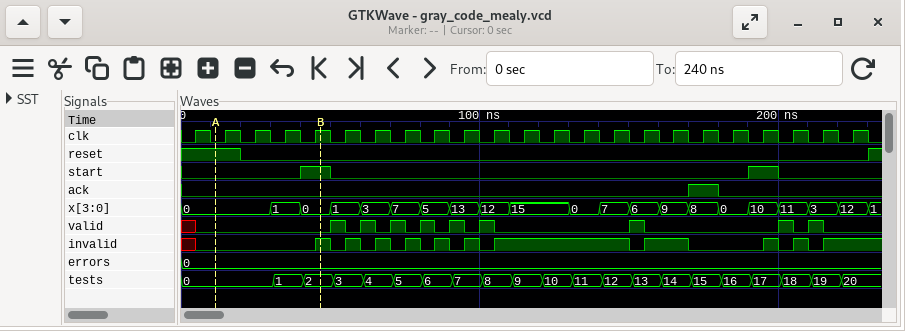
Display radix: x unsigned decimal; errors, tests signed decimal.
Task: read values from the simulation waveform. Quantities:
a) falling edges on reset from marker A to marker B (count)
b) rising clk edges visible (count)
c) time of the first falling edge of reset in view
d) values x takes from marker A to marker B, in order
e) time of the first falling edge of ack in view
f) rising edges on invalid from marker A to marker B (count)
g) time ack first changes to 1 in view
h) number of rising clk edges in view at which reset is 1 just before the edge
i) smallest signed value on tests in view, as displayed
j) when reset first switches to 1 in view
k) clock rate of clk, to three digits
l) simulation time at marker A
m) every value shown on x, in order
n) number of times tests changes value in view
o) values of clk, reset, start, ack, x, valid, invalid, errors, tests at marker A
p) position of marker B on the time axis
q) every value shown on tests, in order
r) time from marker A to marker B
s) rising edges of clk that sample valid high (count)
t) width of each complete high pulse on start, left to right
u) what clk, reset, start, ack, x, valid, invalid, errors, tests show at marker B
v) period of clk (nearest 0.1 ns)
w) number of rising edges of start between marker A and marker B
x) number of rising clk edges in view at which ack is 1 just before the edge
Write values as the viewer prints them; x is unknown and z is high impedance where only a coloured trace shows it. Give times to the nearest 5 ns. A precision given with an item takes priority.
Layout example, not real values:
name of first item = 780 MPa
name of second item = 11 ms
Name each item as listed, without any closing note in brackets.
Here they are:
falling edges on reset from marker A to marker B = 1
rising clk edges visible = 23
time of the first falling edge of reset in view = 20 ns
values x takes from marker A to marker B, in order = 0, 1, 0
time of the first falling edge of ack in view = 180 ns
rising edges on invalid from marker A to marker B = 1
time ack first changes to 1 in view = 170 ns
number of rising clk edges in view at which reset is 1 just before the edge = 2
smallest signed value on tests in view, as displayed = 0
when reset first switches to 1 in view = 230 ns
clock rate of clk, to three digits = 100 MHz
simulation time at marker A = 10 ns
every value shown on x, in order = 0, 1, 0, 1, 3, 7, 5, 13, 12, 15, 0, 7, 6, 9, 8, 0, 10, 11, 3, 12, 1
number of times tests changes value in view = 20
values of clk, reset, start, ack, x, valid, invalid, errors, tests at marker A = clk=0, reset=1, start=0, ack=0, x=0, valid=0, invalid=0, errors=0, tests=0
position of marker B on the time axis = 45 ns
every value shown on tests, in order = 0, 1, 2, 3, 4, 5, 6, 7, 8, 9, 10, 11, 12, 13, 14, 15, 16, 17, 18, 19, 20
time from marker A to marker B = 35 ns
rising edges of clk that sample valid high = 9
width of each complete high pulse on start, left to right = 10 ns, 10 ns
what clk, reset, start, ack, x, valid, invalid, errors, tests show at marker B = clk=1, reset=0, start=1, ack=0, x=0, valid=0, invalid=1, errors=0, tests=2
period of clk = 10 ns
number of rising edges of start between marker A and marker B = 1
number of rising clk edges in view at which ack is 1 just before the edge = 1
